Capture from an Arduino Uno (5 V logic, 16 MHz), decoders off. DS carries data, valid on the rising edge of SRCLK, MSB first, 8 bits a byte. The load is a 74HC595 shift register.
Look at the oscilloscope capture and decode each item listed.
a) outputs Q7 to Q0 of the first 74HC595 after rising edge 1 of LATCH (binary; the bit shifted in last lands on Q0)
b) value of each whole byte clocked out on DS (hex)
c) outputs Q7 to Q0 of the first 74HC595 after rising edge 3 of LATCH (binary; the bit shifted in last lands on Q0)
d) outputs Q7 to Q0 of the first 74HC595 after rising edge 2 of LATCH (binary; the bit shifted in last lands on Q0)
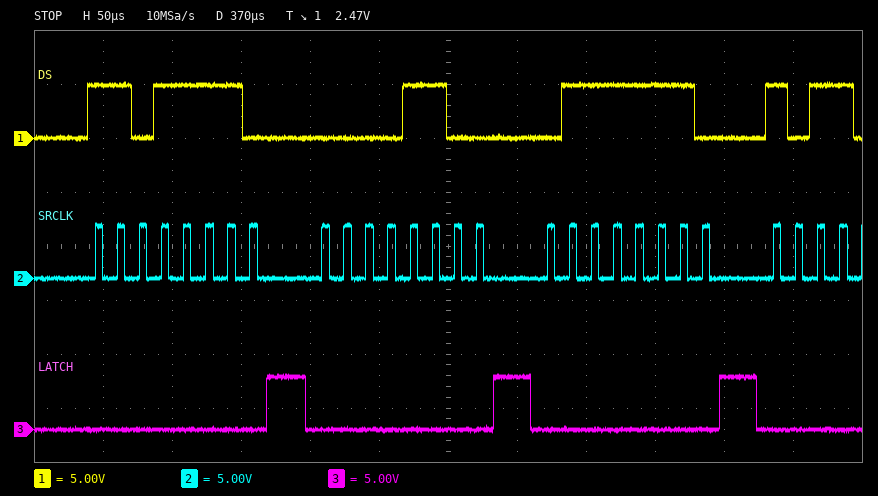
11011110
0xDE 0x0C 0x7E
01111110
00001100
